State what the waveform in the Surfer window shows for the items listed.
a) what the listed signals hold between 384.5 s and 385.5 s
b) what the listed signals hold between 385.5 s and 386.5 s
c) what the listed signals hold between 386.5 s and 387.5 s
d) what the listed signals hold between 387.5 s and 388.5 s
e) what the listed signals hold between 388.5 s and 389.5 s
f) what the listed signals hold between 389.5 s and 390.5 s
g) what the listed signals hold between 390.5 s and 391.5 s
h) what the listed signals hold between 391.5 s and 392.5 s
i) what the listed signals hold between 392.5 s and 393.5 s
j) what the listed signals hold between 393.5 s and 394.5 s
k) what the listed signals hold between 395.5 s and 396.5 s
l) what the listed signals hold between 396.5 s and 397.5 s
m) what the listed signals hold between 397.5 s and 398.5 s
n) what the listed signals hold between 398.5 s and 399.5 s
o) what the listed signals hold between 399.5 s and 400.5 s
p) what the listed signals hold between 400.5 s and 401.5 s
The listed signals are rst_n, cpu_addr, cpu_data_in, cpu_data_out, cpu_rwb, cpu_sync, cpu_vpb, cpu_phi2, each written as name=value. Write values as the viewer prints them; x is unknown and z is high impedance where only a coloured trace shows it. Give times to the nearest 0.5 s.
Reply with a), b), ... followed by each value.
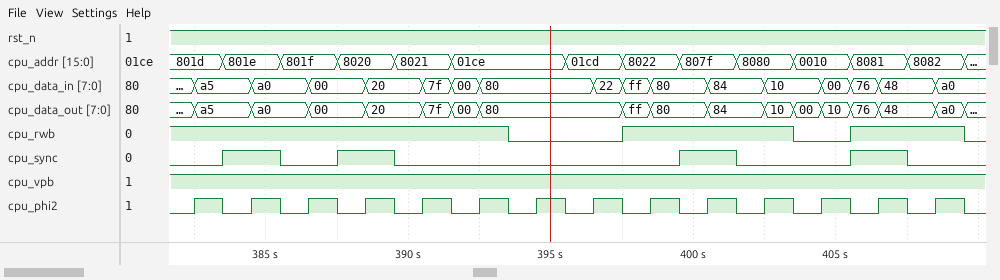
a) rst_n=1, cpu_addr=801e, cpu_data_in=a0, cpu_data_out=a0, cpu_rwb=1, cpu_sync=1, cpu_vpb=1, cpu_phi2=1
b) rst_n=1, cpu_addr=801f, cpu_data_in=a0, cpu_data_out=a0, cpu_rwb=1, cpu_sync=0, cpu_vpb=1, cpu_phi2=0
c) rst_n=1, cpu_addr=801f, cpu_data_in=00, cpu_data_out=00, cpu_rwb=1, cpu_sync=0, cpu_vpb=1, cpu_phi2=1
d) rst_n=1, cpu_addr=8020, cpu_data_in=00, cpu_data_out=00, cpu_rwb=1, cpu_sync=1, cpu_vpb=1, cpu_phi2=0
e) rst_n=1, cpu_addr=8020, cpu_data_in=20, cpu_data_out=20, cpu_rwb=1, cpu_sync=1, cpu_vpb=1, cpu_phi2=1
f) rst_n=1, cpu_addr=8021, cpu_data_in=20, cpu_data_out=20, cpu_rwb=1, cpu_sync=0, cpu_vpb=1, cpu_phi2=0
g) rst_n=1, cpu_addr=8021, cpu_data_in=7f, cpu_data_out=7f, cpu_rwb=1, cpu_sync=0, cpu_vpb=1, cpu_phi2=1
h) rst_n=1, cpu_addr=01ce, cpu_data_in=00, cpu_data_out=00, cpu_rwb=1, cpu_sync=0, cpu_vpb=1, cpu_phi2=0
i) rst_n=1, cpu_addr=01ce, cpu_data_in=80, cpu_data_out=80, cpu_rwb=1, cpu_sync=0, cpu_vpb=1, cpu_phi2=1
j) rst_n=1, cpu_addr=01ce, cpu_data_in=80, cpu_data_out=80, cpu_rwb=0, cpu_sync=0, cpu_vpb=1, cpu_phi2=0
k) rst_n=1, cpu_addr=01cd, cpu_data_in=80, cpu_data_out=80, cpu_rwb=0, cpu_sync=0, cpu_vpb=1, cpu_phi2=0
l) rst_n=1, cpu_addr=01cd, cpu_data_in=22, cpu_data_out=80, cpu_rwb=0, cpu_sync=0, cpu_vpb=1, cpu_phi2=1
m) rst_n=1, cpu_addr=8022, cpu_data_in=ff, cpu_data_out=ff, cpu_rwb=1, cpu_sync=0, cpu_vpb=1, cpu_phi2=0
n) rst_n=1, cpu_addr=8022, cpu_data_in=80, cpu_data_out=80, cpu_rwb=1, cpu_sync=0, cpu_vpb=1, cpu_phi2=1
o) rst_n=1, cpu_addr=807f, cpu_data_in=80, cpu_data_out=80, cpu_rwb=1, cpu_sync=1, cpu_vpb=1, cpu_phi2=0
p) rst_n=1, cpu_addr=807f, cpu_data_in=84, cpu_data_out=84, cpu_rwb=1, cpu_sync=1, cpu_vpb=1, cpu_phi2=1
